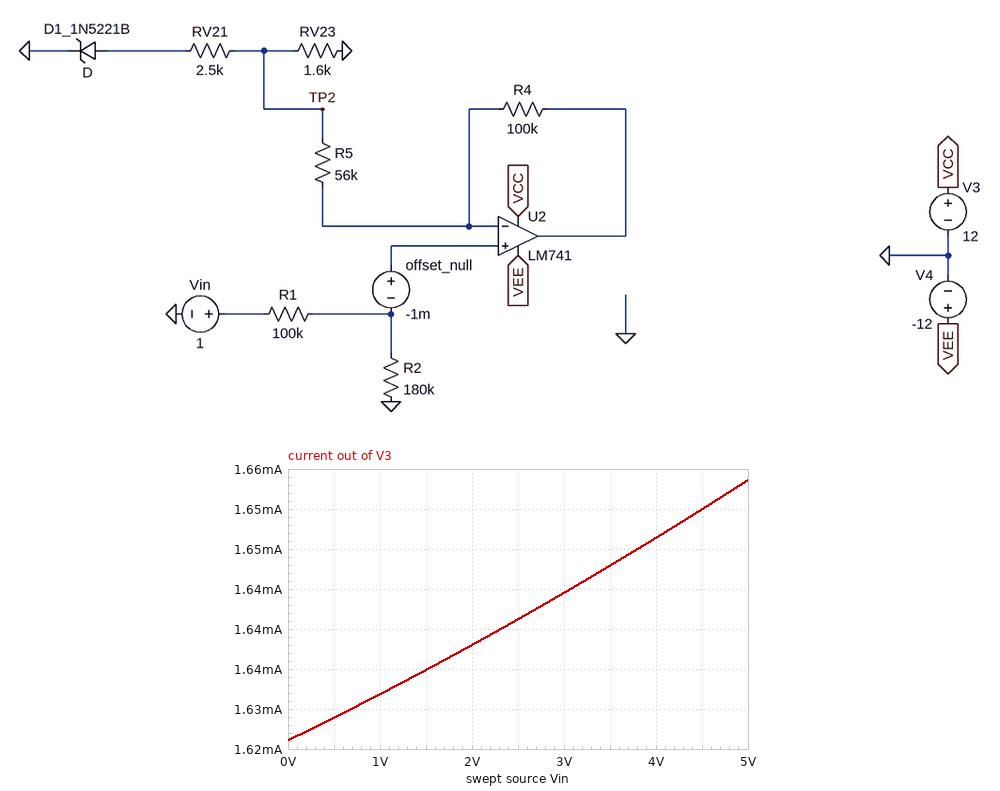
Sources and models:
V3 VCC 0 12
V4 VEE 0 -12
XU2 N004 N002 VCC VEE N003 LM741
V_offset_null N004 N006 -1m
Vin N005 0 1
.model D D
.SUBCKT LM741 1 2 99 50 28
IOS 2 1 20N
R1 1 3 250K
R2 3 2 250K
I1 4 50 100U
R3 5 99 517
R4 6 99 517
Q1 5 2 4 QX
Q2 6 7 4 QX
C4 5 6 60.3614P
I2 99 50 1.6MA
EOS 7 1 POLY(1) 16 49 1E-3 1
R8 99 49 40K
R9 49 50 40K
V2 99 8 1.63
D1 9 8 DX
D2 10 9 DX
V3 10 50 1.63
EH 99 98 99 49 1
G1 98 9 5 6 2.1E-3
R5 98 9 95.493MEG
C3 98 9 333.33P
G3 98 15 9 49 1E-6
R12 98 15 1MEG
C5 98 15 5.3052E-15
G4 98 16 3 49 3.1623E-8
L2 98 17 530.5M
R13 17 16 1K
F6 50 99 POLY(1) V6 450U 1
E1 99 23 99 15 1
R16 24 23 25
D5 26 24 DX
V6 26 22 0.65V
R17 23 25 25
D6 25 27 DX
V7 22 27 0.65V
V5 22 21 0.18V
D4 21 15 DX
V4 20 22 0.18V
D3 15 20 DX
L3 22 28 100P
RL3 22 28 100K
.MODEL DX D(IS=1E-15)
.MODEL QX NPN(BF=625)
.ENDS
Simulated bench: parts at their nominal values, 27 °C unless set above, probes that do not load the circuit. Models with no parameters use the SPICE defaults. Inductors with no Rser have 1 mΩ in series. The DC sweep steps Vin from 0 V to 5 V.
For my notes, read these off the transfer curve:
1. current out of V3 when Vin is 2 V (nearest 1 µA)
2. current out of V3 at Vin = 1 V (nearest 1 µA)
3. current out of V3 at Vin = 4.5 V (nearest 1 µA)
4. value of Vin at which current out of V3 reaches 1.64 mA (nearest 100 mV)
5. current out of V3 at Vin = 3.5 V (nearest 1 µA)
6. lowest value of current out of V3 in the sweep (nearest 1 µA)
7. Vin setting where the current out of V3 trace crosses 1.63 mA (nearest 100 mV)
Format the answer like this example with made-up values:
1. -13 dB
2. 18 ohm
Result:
1. 1.638 mA
2. 1.632 mA
3. 1.655 mA
4. 2.3 V
5. 1.648 mA
6. 1.626 mA
7. 700 mV
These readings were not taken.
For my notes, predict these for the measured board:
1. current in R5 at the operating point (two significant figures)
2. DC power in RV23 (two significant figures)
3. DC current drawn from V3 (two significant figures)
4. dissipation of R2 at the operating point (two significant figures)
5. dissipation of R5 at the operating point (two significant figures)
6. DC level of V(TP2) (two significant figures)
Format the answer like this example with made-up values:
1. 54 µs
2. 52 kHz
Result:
1. 11 µA
2. 200 nW
3. 1.6 mA
4. 2.3 µW
5. 6.9 µW
6. 18 mV
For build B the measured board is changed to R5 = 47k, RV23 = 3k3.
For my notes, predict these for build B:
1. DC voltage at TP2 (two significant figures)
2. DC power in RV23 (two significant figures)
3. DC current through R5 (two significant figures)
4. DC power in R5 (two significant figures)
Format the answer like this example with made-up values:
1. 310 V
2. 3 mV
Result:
1. 42 mV
2. 530 nW
3. 13 µA
4. 7.6 µW
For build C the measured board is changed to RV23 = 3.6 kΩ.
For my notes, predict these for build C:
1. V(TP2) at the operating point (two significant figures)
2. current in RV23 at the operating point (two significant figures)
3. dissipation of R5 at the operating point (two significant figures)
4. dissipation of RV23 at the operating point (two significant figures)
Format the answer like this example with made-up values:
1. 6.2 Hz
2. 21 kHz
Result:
1. 39 mV
2. 11 µA
3. 6.4 µW
4. 410 nW
